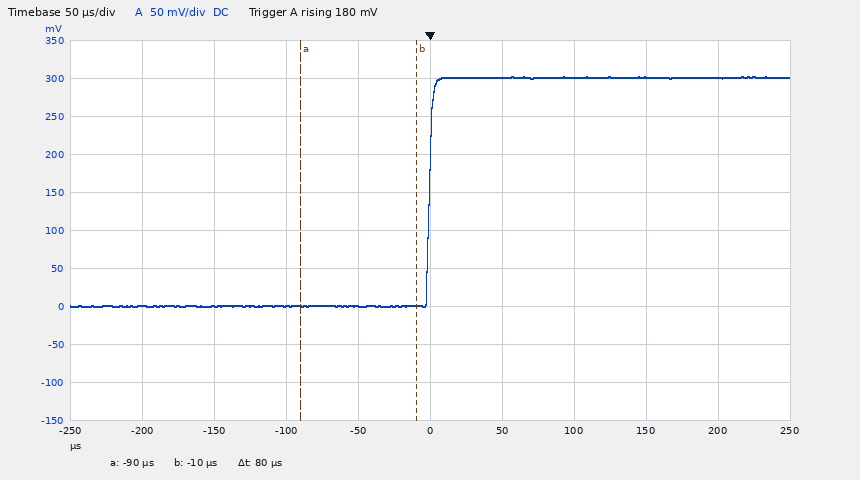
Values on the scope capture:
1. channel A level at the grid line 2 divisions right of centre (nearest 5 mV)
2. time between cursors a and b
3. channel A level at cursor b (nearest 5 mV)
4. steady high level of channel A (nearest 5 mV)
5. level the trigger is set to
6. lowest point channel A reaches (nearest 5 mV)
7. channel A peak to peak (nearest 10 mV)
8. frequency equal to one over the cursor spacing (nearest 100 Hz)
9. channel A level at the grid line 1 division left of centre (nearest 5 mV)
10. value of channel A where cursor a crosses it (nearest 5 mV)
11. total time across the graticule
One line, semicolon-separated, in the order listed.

300 mV; 80 µs; 0 mV; 300 mV; 180 mV; 0 mV; 300 mV; 12.5 kHz; 0 mV; 0 mV; 500 µs
